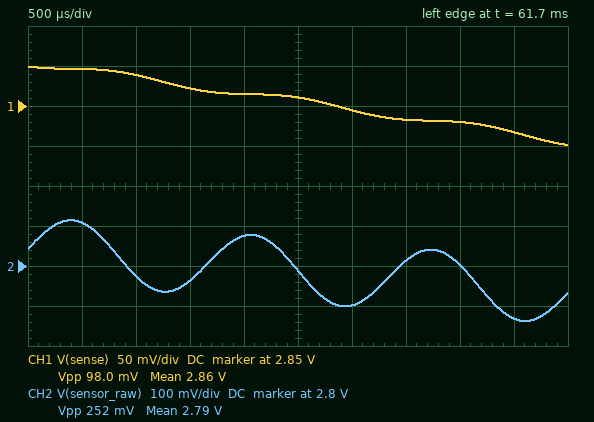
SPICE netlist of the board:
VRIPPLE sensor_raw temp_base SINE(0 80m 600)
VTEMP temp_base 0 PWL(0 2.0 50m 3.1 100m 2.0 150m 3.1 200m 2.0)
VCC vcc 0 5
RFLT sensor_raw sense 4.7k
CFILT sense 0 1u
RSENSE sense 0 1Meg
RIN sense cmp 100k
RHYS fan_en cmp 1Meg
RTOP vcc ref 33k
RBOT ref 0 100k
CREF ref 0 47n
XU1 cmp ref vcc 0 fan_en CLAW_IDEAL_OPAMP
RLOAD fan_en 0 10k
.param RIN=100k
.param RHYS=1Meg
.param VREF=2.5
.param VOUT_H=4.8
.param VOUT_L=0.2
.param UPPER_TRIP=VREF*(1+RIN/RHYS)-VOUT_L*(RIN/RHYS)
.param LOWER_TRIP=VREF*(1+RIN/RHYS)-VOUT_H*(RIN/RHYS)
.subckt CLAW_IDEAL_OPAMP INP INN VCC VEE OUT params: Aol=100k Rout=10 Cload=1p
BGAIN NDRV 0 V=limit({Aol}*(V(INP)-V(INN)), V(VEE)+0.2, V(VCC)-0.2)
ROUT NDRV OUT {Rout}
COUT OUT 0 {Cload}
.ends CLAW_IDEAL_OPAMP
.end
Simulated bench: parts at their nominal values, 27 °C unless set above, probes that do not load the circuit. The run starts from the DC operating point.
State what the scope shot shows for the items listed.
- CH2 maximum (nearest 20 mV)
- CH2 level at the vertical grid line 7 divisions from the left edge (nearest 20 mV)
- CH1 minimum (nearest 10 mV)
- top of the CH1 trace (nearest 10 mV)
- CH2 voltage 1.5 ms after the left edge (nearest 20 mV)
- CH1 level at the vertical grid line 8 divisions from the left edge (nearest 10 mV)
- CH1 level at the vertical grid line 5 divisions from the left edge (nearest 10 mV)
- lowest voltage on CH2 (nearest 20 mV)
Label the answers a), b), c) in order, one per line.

a) 2.92 V
b) 2.82 V
c) 2.80 V
d) 2.90 V
e) 2.76 V
f) 2.83 V
g) 2.86 V
h) 2.66 V
